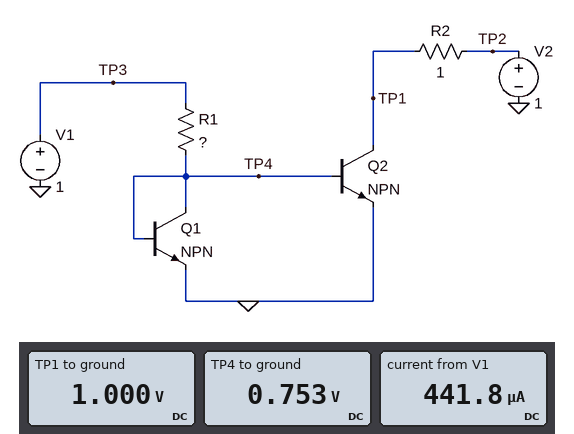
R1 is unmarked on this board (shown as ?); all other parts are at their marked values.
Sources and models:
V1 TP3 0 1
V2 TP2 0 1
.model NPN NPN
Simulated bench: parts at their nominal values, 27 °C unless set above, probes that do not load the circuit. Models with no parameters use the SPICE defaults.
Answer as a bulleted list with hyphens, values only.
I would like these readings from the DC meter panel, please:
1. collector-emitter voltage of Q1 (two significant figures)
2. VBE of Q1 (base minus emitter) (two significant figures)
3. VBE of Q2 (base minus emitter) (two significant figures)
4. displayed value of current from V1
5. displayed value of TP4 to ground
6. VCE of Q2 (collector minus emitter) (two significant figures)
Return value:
- 750 mV
- 750 mV
- 750 mV
- 441.8 µA
- 0.753 V
- 1.0 V
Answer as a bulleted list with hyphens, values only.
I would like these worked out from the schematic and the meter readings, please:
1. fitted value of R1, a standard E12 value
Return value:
- 560 Ω
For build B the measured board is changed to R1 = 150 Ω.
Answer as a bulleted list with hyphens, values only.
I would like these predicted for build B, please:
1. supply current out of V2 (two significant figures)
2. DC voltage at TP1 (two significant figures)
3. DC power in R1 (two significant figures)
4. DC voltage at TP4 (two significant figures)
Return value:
- 1.4 mA
- 1.0 V
- 310 µW
- 780 mV
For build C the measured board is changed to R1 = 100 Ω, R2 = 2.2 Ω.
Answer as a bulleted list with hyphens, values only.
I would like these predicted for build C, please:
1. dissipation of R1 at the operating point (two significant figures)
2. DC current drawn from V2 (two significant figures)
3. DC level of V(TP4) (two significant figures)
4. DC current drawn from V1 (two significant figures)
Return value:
- 430 µW
- 2.0 mA
- 790 mV
- 2.1 mA
